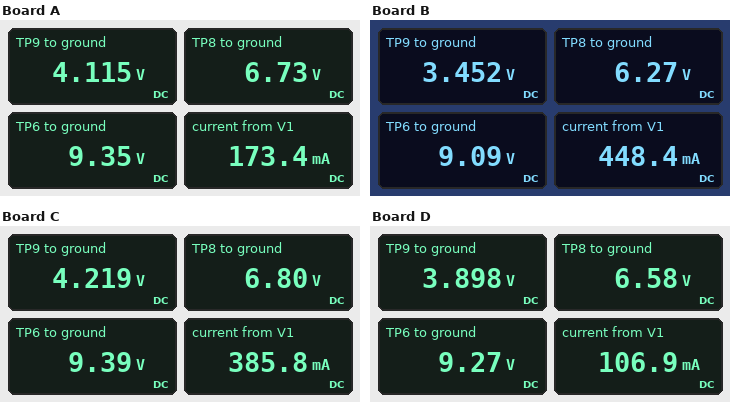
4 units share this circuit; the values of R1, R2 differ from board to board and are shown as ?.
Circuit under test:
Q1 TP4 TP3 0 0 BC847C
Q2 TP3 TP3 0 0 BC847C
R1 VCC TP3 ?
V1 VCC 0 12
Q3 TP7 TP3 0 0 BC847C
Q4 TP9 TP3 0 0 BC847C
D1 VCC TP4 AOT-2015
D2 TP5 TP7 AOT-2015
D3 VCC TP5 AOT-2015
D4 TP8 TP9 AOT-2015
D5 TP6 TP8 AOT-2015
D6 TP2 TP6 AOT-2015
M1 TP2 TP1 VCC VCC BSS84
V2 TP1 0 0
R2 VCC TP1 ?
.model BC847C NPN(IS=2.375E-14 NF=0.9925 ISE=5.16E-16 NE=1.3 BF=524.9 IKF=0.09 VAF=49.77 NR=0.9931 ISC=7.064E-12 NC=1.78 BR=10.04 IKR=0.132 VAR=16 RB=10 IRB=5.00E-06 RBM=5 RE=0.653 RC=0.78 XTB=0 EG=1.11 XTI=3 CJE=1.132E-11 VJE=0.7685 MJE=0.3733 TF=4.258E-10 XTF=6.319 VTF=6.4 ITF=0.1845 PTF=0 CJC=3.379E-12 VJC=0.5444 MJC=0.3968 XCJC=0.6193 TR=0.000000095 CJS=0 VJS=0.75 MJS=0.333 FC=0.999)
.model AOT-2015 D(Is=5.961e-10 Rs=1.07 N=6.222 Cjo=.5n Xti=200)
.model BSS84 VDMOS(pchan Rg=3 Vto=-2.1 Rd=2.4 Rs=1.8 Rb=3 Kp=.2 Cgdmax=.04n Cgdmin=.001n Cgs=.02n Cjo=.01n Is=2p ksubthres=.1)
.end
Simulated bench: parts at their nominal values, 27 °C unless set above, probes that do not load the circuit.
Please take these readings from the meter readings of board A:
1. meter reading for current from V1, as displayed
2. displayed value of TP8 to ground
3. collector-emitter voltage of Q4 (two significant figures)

173.4 mA
6.73 V
4.1 V
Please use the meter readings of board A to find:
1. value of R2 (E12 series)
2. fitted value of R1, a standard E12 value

82 Ω
1.8 kΩ
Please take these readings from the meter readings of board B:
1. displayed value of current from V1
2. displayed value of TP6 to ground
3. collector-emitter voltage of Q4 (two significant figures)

448.4 mA
9.09 V
3.5 V
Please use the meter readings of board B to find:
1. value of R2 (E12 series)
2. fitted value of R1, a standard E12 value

33 Ω
560 Ω
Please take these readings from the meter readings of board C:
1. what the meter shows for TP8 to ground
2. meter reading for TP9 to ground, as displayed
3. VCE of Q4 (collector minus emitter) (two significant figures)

6.80 V
4.219 V
4.2 V
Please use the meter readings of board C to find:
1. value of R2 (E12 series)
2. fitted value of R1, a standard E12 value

33 Ω
2.2 kΩ
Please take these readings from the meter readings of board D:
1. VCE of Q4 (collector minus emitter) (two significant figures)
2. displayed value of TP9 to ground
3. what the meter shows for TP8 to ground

3.9 V
3.898 V
6.58 V
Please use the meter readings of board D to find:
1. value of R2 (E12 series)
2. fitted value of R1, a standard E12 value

180 Ω
1.2 kΩ
